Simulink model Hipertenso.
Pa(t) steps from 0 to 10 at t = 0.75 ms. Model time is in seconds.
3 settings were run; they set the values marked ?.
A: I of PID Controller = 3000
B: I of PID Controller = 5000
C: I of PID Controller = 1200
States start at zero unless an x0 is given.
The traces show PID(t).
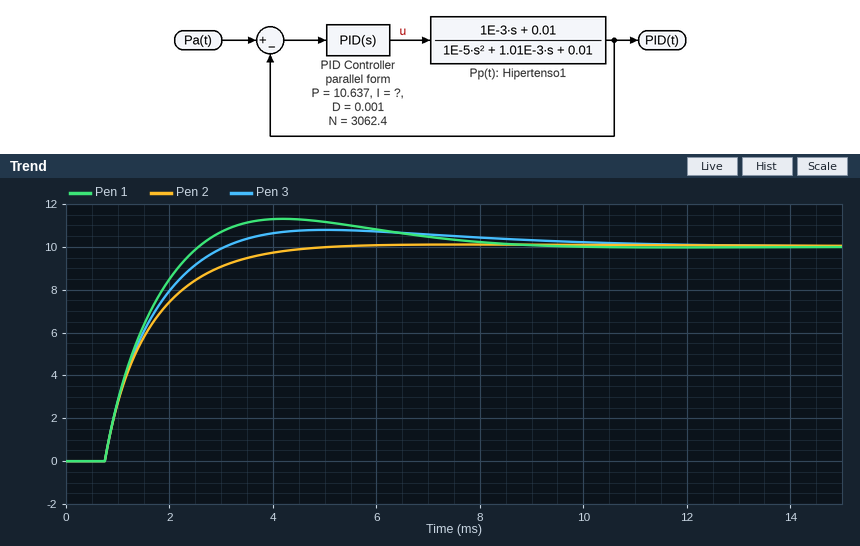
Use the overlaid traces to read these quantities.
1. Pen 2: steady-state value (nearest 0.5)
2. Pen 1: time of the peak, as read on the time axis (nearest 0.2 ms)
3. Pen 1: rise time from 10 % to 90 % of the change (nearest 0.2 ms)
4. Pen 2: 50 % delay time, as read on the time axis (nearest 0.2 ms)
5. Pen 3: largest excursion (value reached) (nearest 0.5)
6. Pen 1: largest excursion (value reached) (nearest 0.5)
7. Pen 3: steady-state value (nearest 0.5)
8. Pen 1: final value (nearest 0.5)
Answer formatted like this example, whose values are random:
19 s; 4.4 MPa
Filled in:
10.0; 4.2 ms; 1.4 ms; 1.4 ms; 11.0; 11.5; 10.0; 10.0
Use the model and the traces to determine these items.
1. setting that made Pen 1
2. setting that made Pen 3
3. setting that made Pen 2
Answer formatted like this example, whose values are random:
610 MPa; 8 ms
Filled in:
B; A; C
